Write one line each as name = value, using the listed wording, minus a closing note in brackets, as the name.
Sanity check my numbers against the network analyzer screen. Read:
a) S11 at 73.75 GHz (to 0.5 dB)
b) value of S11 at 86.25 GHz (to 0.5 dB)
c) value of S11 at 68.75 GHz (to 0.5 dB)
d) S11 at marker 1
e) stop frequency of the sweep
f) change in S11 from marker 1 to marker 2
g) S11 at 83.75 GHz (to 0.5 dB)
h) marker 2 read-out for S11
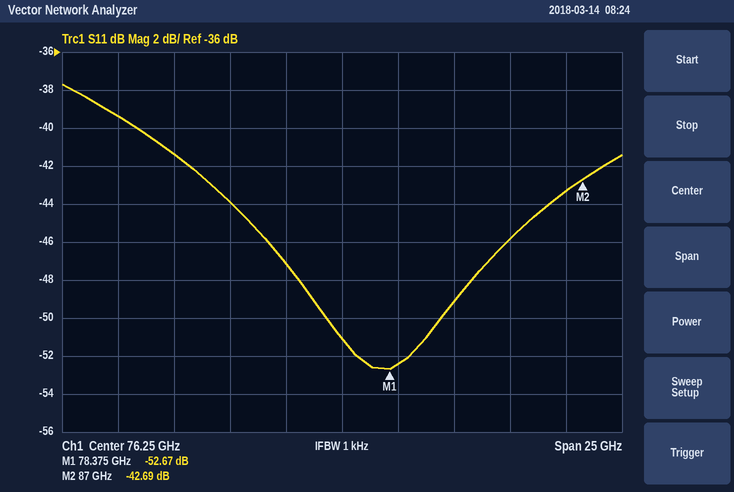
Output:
S11 at 73.75 GHz = -47.0 dB
value of S11 at 86.25 GHz = -43.5 dB
value of S11 at 68.75 GHz = -41.5 dB
S11 at marker 1 = -52.67 dB
stop frequency of the sweep = 88.75 GHz
change in S11 from marker 1 to marker 2 = 9.98 dB
S11 at 83.75 GHz = -46.0 dB
marker 2 read-out for S11 = -42.69 dB
